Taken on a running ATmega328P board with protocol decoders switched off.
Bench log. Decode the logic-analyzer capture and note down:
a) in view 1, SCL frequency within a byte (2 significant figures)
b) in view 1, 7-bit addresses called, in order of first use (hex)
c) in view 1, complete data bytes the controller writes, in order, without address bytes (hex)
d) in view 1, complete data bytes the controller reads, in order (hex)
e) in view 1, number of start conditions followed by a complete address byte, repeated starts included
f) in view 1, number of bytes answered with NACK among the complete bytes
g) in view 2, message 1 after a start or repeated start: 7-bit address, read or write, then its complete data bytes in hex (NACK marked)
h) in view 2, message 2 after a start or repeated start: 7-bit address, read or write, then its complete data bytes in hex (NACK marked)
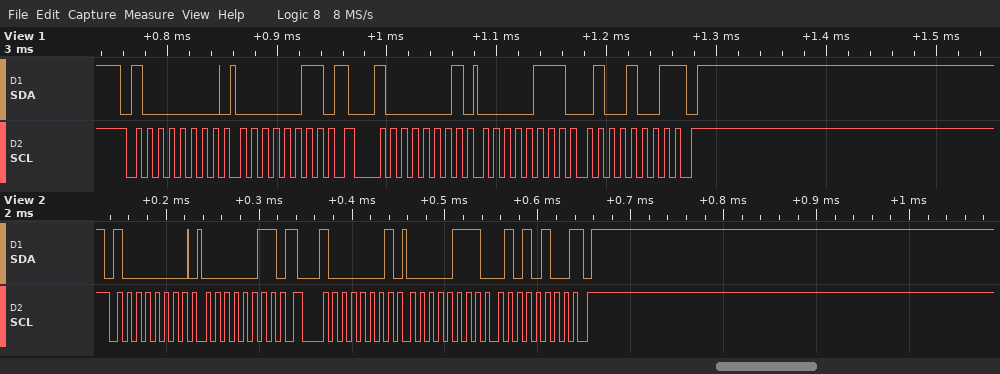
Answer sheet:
100 kHz
0x40
03
07 49
2
1
0x40 write: 03
0x40 read: 07 54 NACK
